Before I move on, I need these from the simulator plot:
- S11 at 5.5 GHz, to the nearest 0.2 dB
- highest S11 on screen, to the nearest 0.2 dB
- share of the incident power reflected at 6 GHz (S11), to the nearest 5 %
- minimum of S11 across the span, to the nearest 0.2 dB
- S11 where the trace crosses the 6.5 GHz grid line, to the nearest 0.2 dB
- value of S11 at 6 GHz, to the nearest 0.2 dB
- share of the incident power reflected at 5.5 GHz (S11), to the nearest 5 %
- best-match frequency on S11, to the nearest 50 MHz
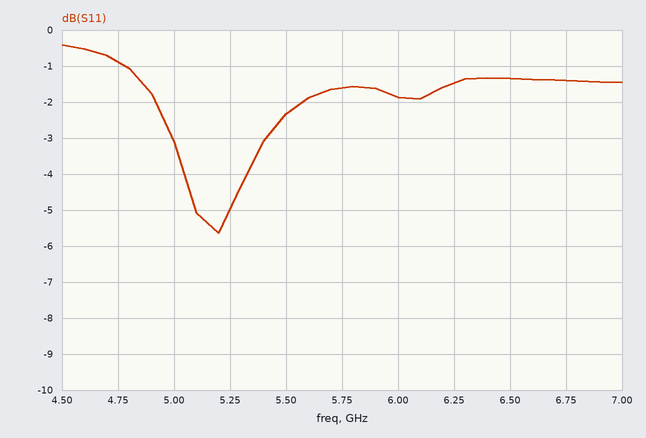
-2.4 dB
-0.4 dB
65 %
-5.6 dB
-1.4 dB
-1.8 dB
60 %
5.20 GHz
